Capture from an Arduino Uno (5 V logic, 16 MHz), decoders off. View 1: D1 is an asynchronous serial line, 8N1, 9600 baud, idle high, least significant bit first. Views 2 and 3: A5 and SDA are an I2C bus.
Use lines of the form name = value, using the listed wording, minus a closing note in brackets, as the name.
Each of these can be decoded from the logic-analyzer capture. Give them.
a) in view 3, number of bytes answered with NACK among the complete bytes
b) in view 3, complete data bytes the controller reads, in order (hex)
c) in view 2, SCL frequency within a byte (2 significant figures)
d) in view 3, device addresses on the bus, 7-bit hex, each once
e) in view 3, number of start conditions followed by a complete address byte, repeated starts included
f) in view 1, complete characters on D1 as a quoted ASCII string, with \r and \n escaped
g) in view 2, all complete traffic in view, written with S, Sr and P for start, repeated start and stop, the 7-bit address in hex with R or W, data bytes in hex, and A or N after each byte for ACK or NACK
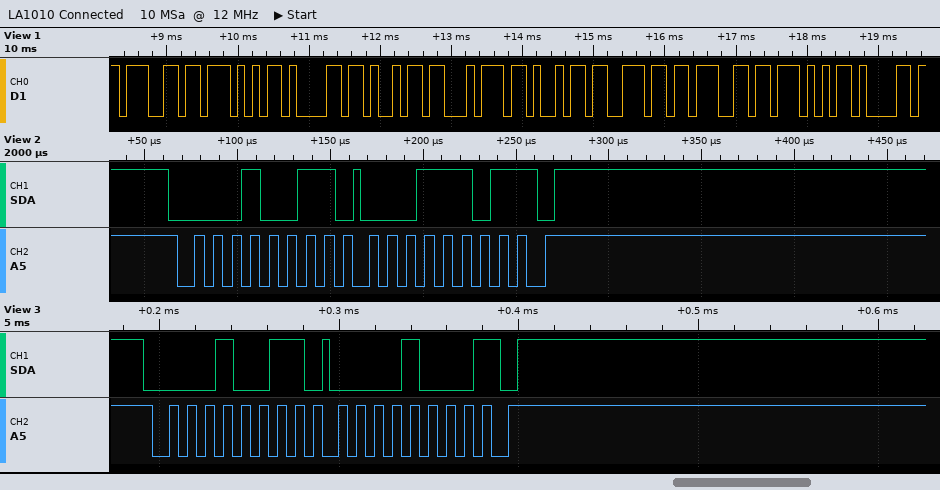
in view 3, number of bytes answered with NACK among the complete bytes = 1
in view 3, complete data bytes the controller reads, in order = 08
in view 2, SCL frequency within a byte = 100 kHz
in view 3, device addresses on the bus, 7-bit hex, each once = 0x09
in view 3, number of start conditions followed by a complete address byte, repeated starts included = 1
in view 1, complete characters on D1 as a quoted ASCII string, with \r and \n escaped = "gWaitingWa"
in view 2, all complete traffic in view, written with S, Sr and P for start, repeated start and stop, the 7-bit address in hex with R or W, data bytes in hex, and A or N after each byte for ACK or NACK = S 09R A 1D N P
